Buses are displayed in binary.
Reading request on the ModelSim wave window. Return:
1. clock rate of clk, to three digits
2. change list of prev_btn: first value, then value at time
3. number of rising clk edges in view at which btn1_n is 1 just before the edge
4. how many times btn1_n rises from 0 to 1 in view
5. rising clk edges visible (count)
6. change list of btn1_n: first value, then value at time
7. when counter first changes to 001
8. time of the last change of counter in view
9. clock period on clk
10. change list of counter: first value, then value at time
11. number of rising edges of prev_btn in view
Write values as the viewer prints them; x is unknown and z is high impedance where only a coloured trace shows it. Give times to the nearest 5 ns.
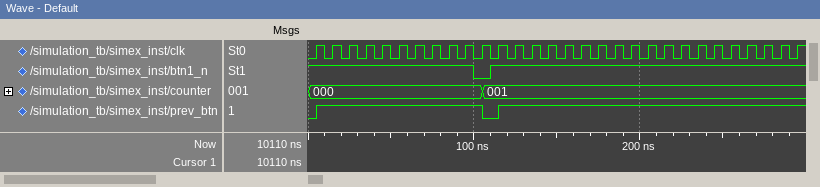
100 MHz
0, 1 at 5 ns, 0 at 105 ns, 1 at 115 ns
29
1
30
1, 0 at 100 ns, 1 at 110 ns
105 ns
105 ns
10 ns
000, 001 at 105 ns
2
